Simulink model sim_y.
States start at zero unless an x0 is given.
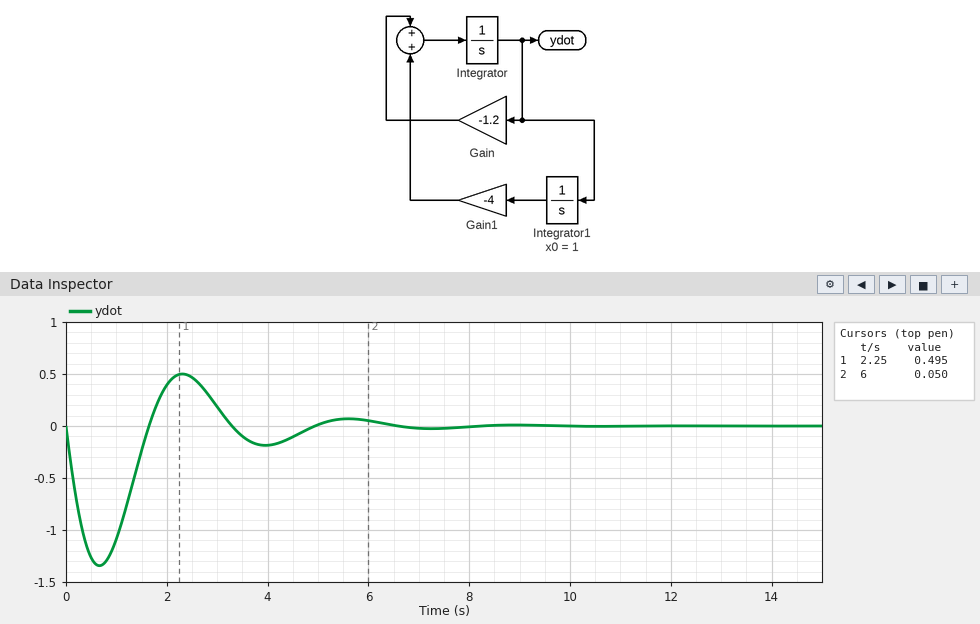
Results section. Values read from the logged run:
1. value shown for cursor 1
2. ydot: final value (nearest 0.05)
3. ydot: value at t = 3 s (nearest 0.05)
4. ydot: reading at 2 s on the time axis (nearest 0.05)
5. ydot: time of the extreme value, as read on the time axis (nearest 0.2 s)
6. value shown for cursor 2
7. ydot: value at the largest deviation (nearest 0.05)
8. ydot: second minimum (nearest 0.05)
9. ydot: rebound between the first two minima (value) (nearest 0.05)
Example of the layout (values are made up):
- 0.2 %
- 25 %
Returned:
- 0.495
- 0.00
- 0.20
- 0.40
- 0.6 s
- 0.050
- -1.35
- -0.20
- 0.50
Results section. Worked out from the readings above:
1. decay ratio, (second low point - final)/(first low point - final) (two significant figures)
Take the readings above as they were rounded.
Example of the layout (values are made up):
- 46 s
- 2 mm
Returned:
- 0.15
